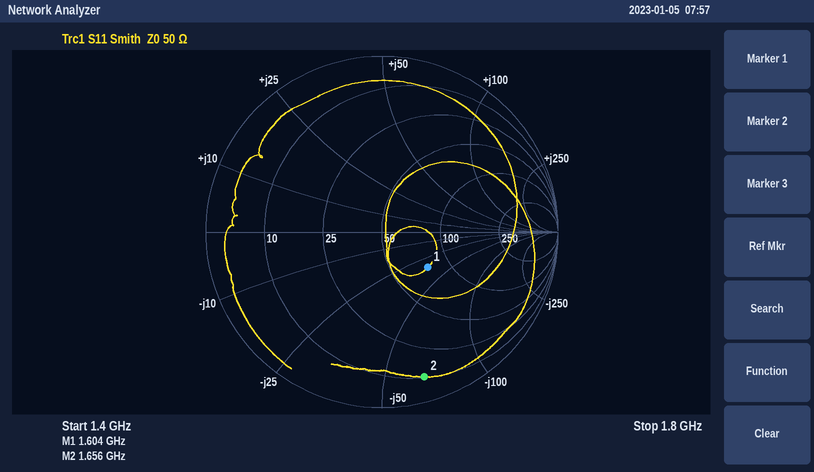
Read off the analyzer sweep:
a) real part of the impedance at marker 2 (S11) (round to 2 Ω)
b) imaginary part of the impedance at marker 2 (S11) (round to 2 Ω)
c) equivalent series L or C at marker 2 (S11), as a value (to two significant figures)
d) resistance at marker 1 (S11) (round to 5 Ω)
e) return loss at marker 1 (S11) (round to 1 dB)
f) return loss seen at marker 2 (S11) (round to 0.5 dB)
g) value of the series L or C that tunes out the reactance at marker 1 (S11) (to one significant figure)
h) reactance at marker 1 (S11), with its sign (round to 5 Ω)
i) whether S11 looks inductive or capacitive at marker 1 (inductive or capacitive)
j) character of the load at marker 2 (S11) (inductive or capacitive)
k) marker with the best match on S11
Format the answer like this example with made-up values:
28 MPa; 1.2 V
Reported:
10 Ω; -66 Ω; 1.5 pF; 75 Ω; 10 dB; 1.5 dB; 3 nH; -35 Ω; capacitive; capacitive; marker 1
